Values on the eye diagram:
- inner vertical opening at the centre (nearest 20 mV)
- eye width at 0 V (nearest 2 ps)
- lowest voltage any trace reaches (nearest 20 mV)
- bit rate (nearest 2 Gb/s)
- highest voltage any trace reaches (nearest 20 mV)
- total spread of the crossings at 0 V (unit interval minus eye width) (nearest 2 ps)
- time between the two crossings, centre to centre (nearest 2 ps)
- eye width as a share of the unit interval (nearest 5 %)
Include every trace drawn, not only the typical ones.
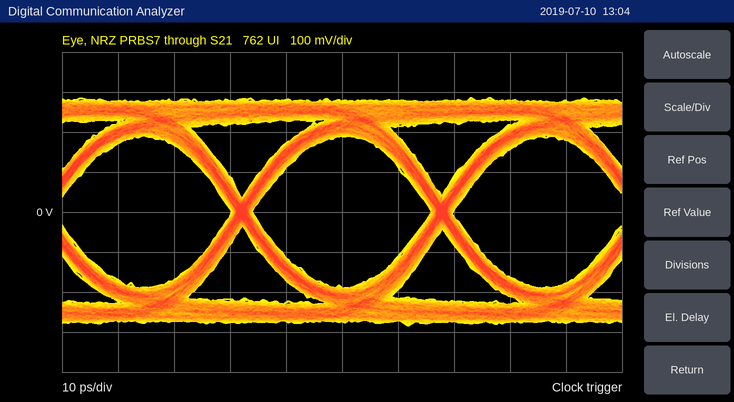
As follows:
380 mV
32 ps
-280 mV
28 Gb/s
280 mV
4 ps
36 ps
90 %
